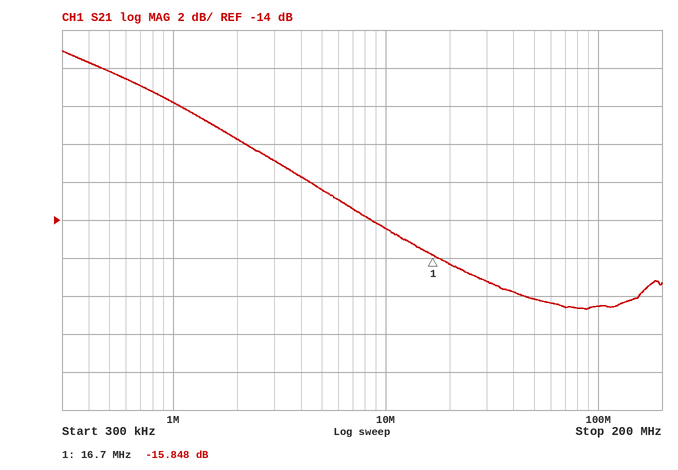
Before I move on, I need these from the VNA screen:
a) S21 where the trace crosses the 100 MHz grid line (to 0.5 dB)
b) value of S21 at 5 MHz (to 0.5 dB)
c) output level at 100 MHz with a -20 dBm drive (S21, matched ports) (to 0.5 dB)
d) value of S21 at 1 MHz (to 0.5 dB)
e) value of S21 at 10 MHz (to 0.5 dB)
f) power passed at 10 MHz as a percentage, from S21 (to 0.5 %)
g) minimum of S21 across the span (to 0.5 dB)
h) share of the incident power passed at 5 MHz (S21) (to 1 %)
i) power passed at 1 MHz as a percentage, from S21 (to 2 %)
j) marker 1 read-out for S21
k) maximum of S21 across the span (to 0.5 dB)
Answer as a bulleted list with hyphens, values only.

- -18.5 dB
- -12.5 dB
- -38.5 dBm
- -8.0 dB
- -14.5 dB
- 3.5 %
- -18.5 dB
- 6 %
- 16 %
- -15.848 dB
- -5.0 dB
